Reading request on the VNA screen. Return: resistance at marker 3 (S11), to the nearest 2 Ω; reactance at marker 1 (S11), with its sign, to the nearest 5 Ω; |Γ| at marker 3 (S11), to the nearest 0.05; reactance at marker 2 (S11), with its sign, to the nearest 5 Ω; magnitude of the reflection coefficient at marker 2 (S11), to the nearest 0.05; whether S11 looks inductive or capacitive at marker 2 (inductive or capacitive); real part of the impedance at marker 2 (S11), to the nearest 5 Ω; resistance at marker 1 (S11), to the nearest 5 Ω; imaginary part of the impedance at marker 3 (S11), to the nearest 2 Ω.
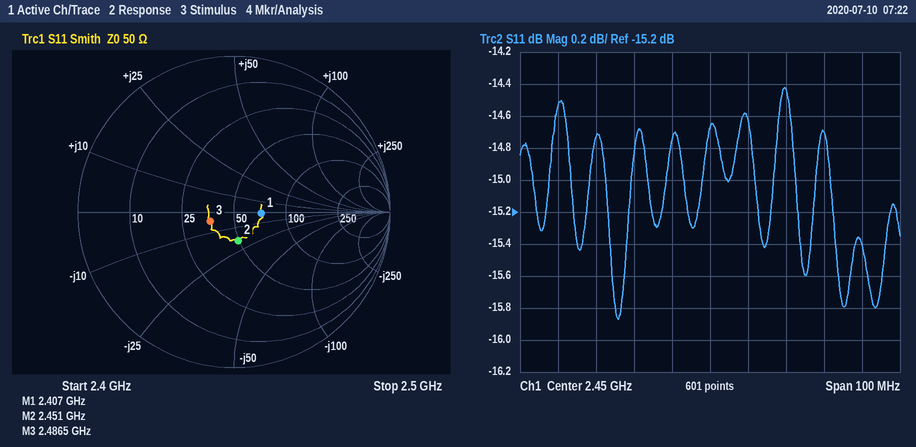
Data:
36 Ω
0 Ω
0.15
-20 Ω
0.20
capacitive
50 Ω
70 Ω
-4 Ω
